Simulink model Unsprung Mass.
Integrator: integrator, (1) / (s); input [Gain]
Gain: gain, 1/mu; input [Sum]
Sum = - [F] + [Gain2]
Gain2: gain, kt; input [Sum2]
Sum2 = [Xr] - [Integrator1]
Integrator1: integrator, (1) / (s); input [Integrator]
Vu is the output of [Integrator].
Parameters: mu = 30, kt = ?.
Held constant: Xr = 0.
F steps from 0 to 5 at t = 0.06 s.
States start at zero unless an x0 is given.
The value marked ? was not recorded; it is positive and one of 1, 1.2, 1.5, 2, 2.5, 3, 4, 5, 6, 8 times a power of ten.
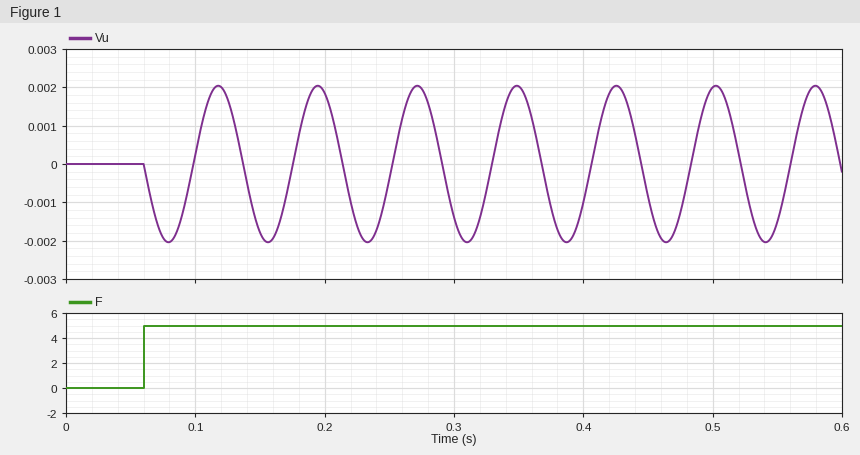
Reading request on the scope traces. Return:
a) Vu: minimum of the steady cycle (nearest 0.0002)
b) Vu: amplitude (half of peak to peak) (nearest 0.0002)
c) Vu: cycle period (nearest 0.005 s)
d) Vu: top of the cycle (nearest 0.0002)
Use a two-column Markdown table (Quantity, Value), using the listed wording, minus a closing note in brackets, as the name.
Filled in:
| Quantity | Value |
|---|---|
| Vu: minimum of the steady cycle | -0.0020 |
| Vu: amplitude (half of peak to peak) | 0.0020 |
| Vu: cycle period | 0.075 s |
| Vu: top of the cycle | 0.0020 |
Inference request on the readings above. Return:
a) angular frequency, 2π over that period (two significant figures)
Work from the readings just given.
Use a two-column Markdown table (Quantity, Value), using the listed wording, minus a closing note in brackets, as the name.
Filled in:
| Quantity | Value |
|---|---|
| angular frequency, 2π over that period | 84 rad/s |
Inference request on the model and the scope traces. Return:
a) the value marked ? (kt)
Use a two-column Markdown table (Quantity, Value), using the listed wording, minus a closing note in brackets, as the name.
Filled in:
| Quantity | Value |
|---|---|
| the value marked ? | 200000 |
